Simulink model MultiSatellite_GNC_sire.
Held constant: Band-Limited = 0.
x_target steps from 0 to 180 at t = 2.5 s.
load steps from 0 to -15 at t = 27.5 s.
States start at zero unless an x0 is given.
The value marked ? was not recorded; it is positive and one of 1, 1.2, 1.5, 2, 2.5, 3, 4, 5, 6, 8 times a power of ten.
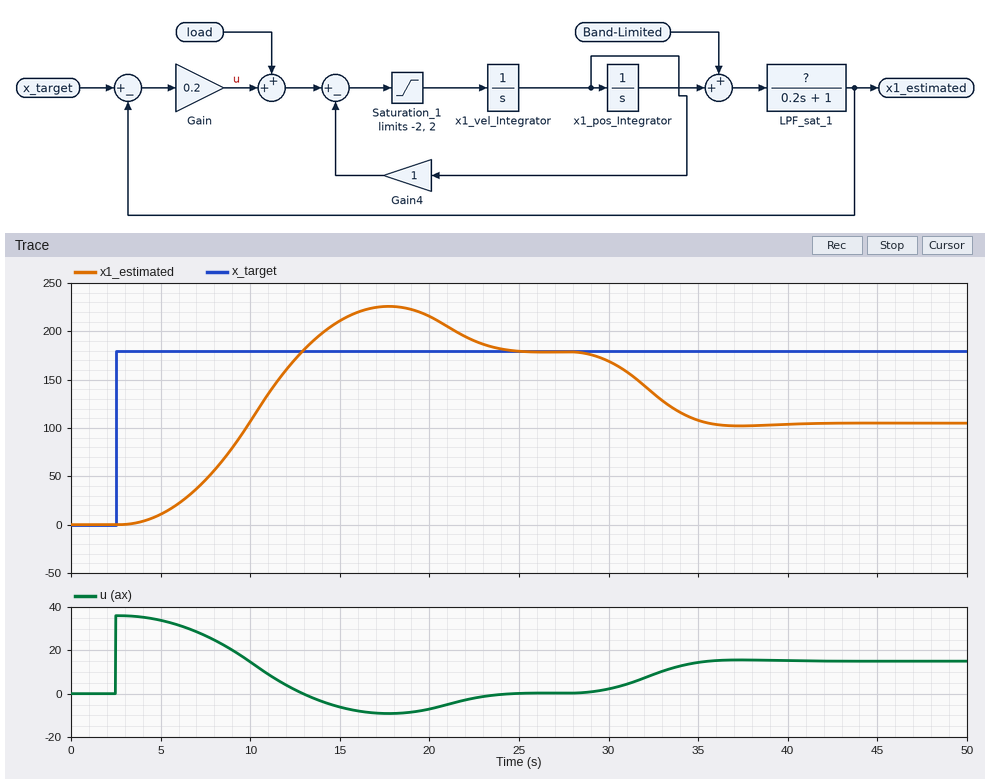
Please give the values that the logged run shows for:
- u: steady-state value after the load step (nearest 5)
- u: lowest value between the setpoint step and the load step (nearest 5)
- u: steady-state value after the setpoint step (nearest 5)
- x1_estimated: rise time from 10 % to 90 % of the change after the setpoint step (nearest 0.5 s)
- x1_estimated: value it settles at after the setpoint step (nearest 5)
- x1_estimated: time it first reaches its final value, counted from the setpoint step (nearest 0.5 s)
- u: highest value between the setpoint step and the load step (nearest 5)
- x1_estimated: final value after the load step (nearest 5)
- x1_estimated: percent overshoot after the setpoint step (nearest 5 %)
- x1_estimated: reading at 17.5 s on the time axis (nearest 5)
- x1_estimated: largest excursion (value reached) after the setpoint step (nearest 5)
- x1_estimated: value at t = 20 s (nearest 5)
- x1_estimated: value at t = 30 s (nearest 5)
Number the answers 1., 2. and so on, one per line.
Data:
1. 15
2. -10
3. 0
4. 6.5 s
5. 180
6. 10.5 s
7. 35
8. 105
9. 25 %
10. 225
11. 225
12. 215
13. 170
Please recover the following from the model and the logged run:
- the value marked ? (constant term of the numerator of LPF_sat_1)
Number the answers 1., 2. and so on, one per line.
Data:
1. 2
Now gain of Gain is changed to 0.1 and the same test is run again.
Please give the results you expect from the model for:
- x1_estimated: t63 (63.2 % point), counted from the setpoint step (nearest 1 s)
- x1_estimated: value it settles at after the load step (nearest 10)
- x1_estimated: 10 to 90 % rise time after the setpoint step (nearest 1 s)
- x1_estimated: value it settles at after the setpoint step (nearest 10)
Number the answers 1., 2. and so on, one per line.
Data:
1. 8 s
2. 30
3. 10 s
4. 180
